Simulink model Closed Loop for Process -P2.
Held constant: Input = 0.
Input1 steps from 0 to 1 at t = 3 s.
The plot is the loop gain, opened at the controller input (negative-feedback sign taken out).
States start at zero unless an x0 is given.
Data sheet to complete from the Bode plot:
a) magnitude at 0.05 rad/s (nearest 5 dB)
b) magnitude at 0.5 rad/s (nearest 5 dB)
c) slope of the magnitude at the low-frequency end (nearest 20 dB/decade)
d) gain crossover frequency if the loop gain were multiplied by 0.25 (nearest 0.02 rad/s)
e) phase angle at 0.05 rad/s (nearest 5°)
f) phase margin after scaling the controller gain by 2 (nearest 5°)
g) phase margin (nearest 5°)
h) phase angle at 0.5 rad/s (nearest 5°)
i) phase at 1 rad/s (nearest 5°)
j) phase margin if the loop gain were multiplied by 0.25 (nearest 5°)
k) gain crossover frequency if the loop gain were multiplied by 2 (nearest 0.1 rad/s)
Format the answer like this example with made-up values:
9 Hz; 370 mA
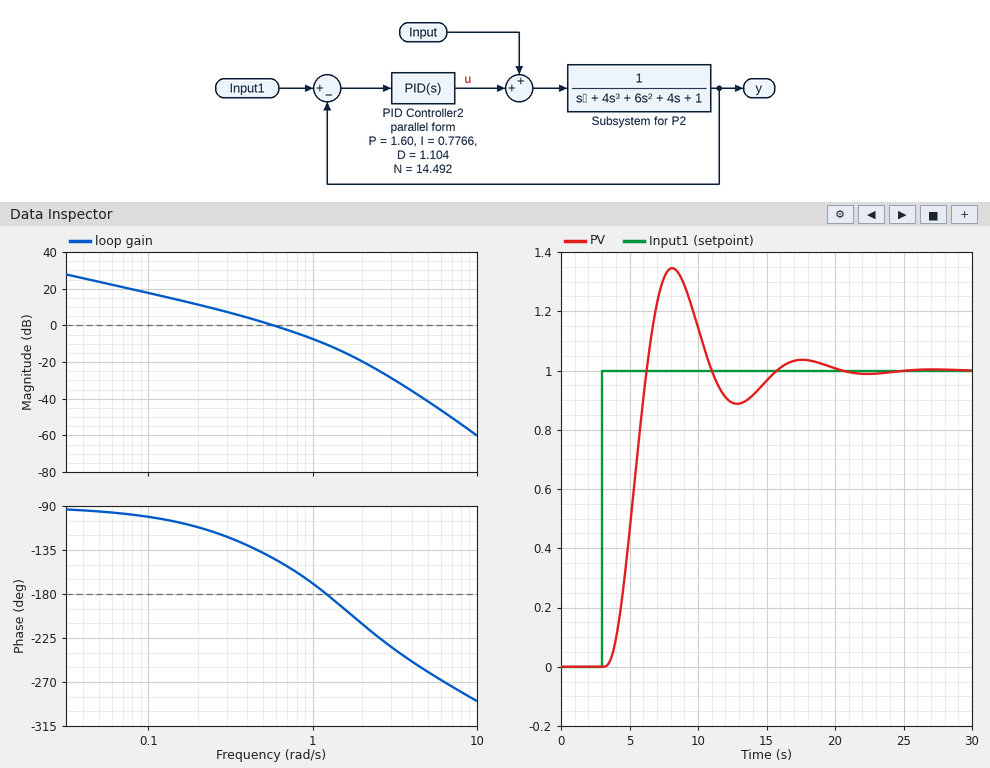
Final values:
25 dB; 0 dB; -20 dB/decade; 0.18 rad/s; -95°; 15°; 35°; -140°; -170°; 70°; 0.9 rad/s
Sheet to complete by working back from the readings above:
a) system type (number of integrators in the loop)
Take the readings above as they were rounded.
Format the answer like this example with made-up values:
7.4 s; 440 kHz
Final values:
1
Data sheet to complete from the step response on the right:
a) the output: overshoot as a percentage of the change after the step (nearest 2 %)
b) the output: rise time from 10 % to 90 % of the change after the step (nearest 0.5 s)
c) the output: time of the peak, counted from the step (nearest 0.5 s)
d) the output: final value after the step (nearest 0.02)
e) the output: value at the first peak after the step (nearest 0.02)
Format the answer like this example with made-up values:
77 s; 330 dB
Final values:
34 %; 2.0 s; 5.0 s; 1.00; 1.34
